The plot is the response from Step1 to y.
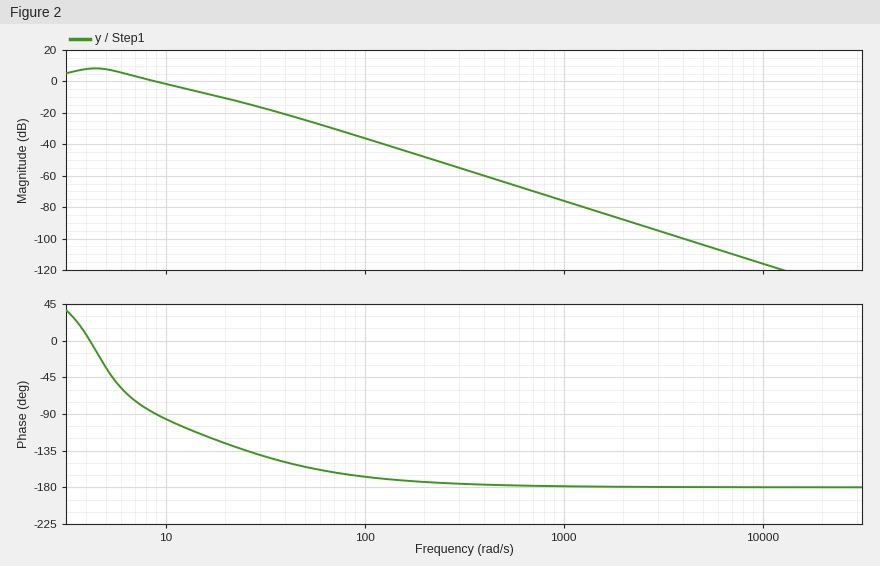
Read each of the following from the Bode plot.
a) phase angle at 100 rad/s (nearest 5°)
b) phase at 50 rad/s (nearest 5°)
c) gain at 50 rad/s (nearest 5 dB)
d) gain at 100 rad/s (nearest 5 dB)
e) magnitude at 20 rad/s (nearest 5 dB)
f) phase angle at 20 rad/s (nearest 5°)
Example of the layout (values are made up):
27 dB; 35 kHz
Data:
-165°; -155°; -25 dB; -35 dB; -10 dB; -125°
